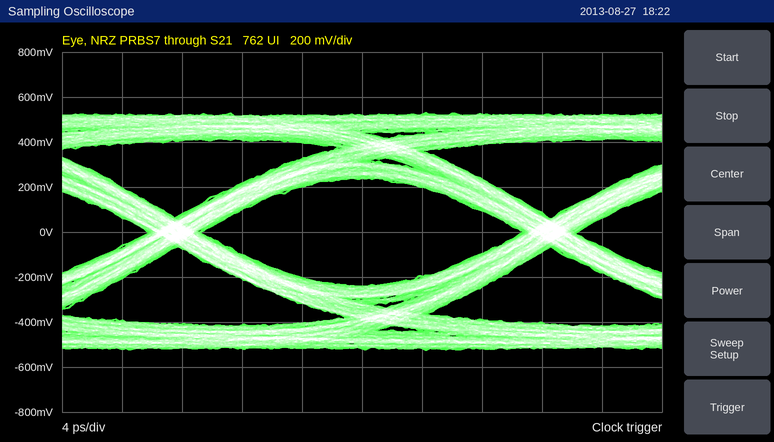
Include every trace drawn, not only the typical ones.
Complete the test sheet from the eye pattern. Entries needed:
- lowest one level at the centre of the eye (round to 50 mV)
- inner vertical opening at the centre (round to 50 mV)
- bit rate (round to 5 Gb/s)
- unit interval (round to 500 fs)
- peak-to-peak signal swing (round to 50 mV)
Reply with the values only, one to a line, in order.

250 mV
500 mV
40 Gb/s
25.0 ps
1.05 V
